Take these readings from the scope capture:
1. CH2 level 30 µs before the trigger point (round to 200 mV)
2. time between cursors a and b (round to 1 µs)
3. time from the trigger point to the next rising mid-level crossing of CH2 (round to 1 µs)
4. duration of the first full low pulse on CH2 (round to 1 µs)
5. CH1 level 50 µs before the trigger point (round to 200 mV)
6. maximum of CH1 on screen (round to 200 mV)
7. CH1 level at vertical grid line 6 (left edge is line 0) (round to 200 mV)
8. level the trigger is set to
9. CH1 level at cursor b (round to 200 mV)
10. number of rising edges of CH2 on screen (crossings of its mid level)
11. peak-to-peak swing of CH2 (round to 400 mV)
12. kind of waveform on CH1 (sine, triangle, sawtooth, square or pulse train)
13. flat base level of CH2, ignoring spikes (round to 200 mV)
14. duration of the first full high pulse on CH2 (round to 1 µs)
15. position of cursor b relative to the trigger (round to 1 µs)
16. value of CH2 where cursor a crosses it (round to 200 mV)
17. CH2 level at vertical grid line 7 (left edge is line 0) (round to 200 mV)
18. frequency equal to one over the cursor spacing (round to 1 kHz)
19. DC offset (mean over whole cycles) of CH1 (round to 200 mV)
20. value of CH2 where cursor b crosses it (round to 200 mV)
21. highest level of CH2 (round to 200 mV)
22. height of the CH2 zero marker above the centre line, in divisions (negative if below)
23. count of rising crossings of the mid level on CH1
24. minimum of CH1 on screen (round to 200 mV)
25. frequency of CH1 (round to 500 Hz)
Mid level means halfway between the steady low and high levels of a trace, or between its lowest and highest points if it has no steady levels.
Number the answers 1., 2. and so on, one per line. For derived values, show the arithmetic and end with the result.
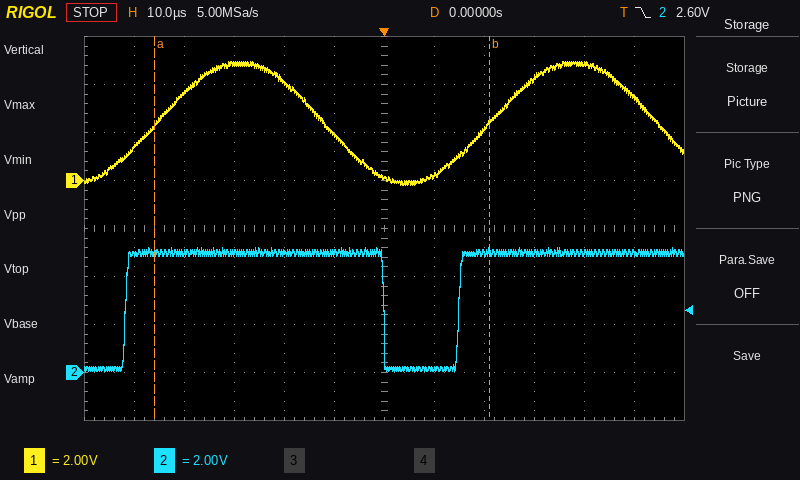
1. 5.0 V
2. 67 µs
3. 15 µs
4. 15 µs
5. 1.4 V
6. 5.0 V
7. 200 mV
8. 2.60 V
9. 2.4 V
10. 2
11. 5.2 V
12. sine
13. 200 mV
14. 52 µs
15. +21 µs
16. 5.0 V
17. 200 mV
18. 1 / 67 µs ≈ 15 kHz
19. (5.0 V + (-200 mV)) / 2 ≈ 2.4 V
20. 5.0 V
21. 5.2 V
22. -3.0 div
23. 2
24. -200 mV
25. 15.0 kHz
